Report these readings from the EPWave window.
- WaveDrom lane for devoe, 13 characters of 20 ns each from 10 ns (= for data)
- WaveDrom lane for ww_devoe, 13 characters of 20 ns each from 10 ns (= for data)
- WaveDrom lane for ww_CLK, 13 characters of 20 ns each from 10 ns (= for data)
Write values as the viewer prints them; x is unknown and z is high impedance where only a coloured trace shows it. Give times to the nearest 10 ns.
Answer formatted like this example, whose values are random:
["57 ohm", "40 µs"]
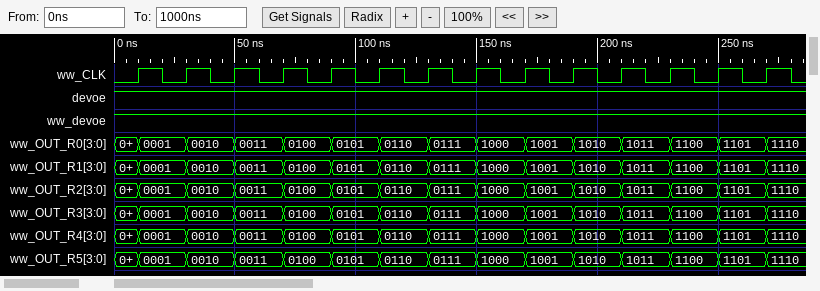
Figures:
["{name: 'devoe', wave: '1............'}", "{name: 'ww_devoe', wave: '1............'}", "{name: 'ww_CLK', wave: 'p............'}"]
